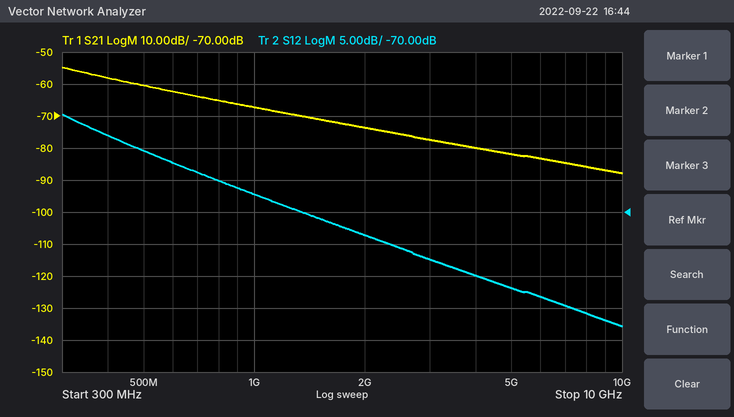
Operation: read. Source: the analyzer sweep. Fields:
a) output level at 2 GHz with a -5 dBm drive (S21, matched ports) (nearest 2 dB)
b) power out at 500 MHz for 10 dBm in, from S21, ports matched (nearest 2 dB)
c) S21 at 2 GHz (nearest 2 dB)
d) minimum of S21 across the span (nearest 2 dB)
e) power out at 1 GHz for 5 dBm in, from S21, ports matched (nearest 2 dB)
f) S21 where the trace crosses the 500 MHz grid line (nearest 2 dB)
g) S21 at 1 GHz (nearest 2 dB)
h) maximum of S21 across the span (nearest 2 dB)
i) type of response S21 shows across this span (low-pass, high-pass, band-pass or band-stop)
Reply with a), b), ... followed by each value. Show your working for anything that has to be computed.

a) -5 dBm + (-74 dB) = -78 dBm
b) 10 dBm + (-60 dB) = -50 dBm
c) -74 dB
d) -88 dB
e) 5 dBm + (-68 dB) = -62 dBm
f) -60 dB
g) -68 dB
h) -54 dB
i) low-pass
